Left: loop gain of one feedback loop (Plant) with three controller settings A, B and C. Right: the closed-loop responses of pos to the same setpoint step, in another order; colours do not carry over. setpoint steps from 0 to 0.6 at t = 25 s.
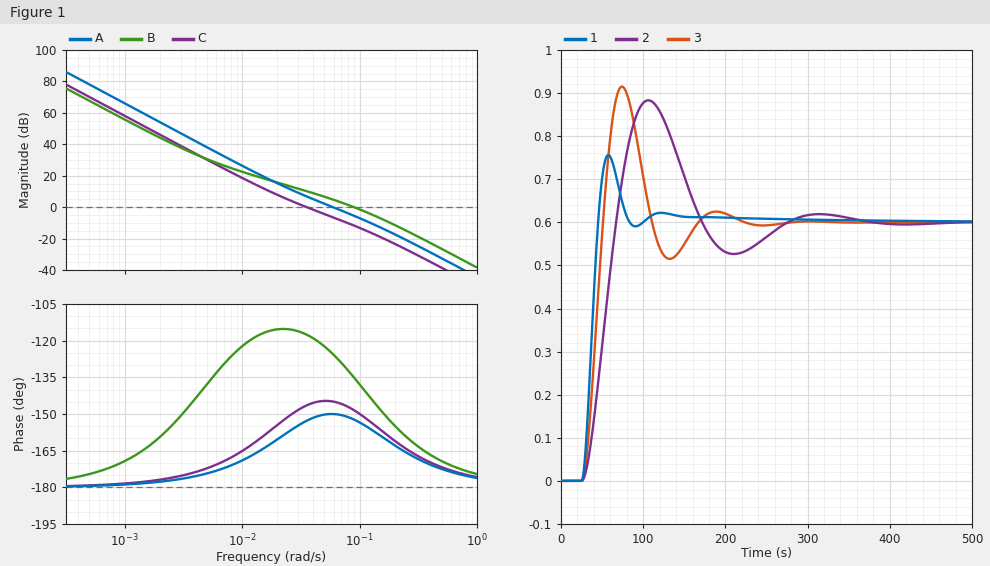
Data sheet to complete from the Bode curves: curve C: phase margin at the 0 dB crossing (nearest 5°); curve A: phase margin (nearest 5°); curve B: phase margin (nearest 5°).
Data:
35°
30°
45°
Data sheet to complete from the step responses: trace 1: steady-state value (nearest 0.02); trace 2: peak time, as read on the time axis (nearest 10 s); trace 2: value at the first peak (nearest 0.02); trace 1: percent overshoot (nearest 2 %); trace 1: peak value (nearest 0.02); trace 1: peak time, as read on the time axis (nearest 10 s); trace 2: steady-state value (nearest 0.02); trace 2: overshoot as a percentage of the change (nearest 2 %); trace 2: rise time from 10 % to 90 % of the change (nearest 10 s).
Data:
0.60
110 s
0.88
26 %
0.76
60 s
0.60
48 %
30 s
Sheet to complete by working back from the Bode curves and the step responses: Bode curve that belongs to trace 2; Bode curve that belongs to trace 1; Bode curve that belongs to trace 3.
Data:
C
B
A
